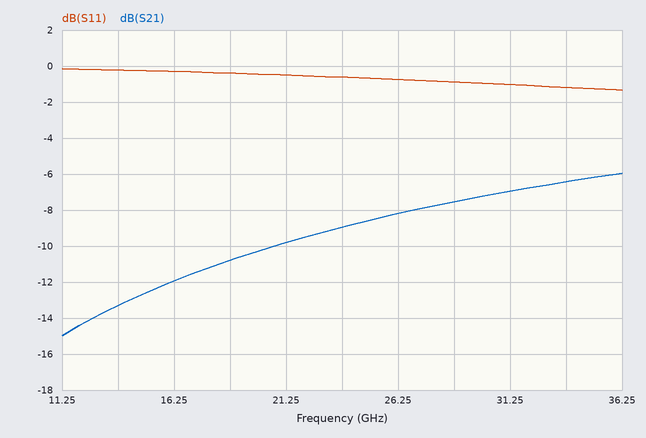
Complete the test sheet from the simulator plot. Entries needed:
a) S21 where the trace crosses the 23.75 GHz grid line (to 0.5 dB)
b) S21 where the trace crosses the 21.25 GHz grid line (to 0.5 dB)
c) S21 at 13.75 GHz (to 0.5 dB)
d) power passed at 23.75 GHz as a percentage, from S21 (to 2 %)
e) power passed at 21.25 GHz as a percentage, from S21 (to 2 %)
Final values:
-9.0 dB
-10.0 dB
-13.5 dB
12 %
10 %
